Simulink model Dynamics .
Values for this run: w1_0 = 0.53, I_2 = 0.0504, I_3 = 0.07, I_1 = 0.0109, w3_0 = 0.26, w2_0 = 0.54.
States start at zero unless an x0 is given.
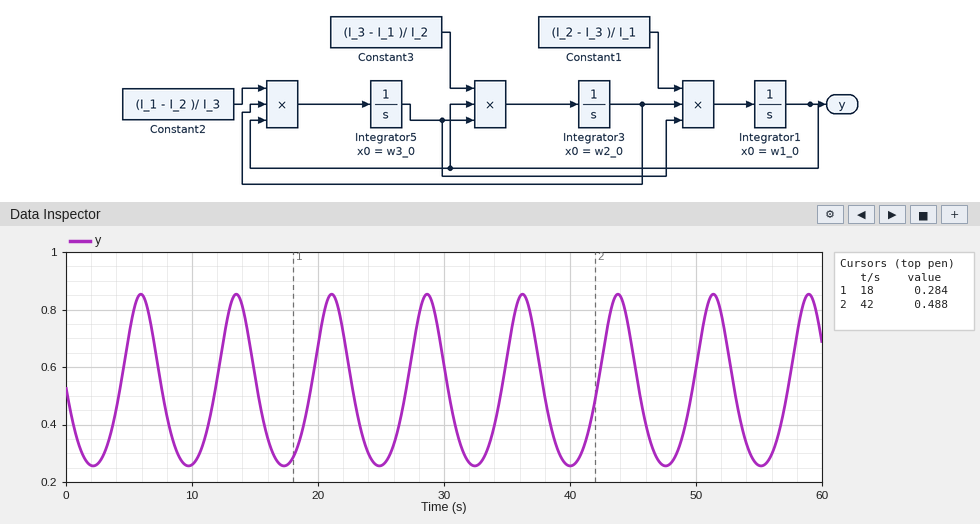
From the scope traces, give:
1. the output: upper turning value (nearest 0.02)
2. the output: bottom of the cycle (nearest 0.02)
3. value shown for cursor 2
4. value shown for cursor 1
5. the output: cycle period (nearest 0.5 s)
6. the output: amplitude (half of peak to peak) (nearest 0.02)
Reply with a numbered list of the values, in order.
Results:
1. 0.86
2. 0.26
3. 0.488
4. 0.284
5. 7.5 s
6. 0.30
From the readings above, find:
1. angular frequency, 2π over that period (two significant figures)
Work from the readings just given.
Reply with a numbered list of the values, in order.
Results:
1. 0.84 rad/s
